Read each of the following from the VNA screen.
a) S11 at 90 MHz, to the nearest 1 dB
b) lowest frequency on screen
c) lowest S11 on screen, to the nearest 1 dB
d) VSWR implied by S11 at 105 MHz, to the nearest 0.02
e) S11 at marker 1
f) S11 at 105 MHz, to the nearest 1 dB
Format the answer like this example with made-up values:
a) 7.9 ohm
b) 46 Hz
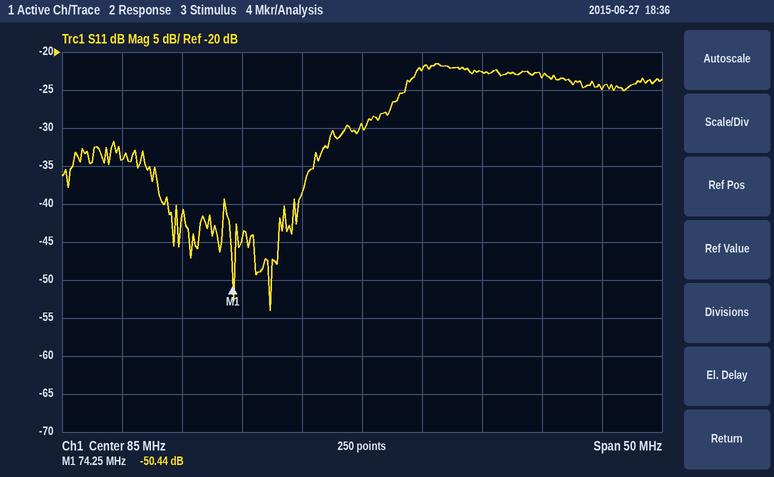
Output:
a) -22 dB
b) 60 MHz
c) -54 dB
d) 1.12
e) -50.44 dB
f) -25 dB
